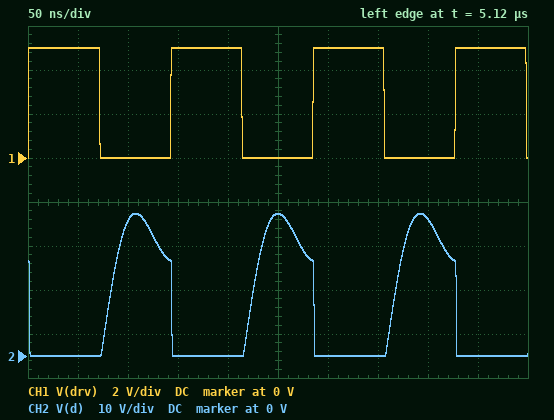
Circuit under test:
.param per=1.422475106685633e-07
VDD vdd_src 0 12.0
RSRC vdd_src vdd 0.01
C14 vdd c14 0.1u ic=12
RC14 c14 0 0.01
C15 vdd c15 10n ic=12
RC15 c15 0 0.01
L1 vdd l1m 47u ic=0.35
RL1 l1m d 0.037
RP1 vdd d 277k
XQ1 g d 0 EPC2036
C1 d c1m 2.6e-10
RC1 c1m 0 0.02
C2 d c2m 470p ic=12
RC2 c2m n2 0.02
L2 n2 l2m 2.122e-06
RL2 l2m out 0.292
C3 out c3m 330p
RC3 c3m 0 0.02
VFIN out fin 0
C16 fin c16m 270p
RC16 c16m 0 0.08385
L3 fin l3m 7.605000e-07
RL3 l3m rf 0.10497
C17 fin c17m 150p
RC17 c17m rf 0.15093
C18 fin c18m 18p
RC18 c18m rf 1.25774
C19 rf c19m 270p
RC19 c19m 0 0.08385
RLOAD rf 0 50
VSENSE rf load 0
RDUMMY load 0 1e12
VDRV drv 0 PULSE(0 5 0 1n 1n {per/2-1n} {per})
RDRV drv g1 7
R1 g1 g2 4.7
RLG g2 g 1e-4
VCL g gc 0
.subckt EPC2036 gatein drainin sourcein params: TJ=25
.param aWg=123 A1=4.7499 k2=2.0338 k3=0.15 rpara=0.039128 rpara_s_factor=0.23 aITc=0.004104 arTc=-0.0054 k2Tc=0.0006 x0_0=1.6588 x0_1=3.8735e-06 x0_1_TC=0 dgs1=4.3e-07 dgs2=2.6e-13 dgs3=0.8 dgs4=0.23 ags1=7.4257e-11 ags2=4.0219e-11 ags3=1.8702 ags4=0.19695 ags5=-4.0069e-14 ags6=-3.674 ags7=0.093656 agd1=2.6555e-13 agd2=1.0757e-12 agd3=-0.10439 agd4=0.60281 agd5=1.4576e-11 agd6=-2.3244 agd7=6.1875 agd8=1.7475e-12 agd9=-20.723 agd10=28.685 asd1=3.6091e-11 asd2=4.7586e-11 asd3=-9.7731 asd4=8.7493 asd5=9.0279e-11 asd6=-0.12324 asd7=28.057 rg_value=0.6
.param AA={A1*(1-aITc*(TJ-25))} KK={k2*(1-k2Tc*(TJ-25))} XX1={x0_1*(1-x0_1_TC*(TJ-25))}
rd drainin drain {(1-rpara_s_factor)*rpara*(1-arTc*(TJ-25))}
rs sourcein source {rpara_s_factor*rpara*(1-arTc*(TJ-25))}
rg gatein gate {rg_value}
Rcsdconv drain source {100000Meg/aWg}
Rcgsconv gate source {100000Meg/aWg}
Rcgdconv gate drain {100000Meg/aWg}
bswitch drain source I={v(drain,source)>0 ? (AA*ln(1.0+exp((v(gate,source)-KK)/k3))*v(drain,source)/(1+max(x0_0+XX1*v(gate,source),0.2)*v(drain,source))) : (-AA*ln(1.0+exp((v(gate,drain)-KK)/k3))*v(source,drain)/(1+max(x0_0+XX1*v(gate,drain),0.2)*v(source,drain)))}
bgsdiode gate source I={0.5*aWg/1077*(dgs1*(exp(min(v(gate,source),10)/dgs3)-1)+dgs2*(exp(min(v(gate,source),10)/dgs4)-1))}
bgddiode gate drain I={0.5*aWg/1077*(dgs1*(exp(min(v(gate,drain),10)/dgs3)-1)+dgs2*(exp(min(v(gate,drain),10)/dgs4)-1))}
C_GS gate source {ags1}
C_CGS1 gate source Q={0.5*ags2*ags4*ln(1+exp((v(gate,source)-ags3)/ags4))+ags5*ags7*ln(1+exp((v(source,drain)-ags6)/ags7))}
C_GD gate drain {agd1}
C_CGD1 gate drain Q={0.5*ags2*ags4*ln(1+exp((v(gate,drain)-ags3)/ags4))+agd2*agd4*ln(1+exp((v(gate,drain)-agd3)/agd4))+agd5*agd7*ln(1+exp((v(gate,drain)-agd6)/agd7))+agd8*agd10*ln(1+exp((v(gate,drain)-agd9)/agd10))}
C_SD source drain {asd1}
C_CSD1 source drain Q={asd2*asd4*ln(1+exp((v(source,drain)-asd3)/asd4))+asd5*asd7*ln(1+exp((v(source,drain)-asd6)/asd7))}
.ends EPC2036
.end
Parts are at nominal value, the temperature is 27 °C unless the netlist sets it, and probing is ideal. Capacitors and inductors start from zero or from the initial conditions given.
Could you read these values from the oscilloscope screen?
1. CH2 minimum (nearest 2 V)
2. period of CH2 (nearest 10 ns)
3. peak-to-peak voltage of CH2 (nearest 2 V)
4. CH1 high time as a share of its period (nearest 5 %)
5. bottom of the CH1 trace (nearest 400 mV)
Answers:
0 V
140 ns
32 V
50 %
0 V
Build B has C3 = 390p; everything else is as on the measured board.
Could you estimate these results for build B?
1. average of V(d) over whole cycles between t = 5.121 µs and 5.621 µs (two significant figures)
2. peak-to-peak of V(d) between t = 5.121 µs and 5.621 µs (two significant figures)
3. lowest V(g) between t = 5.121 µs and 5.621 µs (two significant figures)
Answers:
12 V
33 V
-9.5 mV
